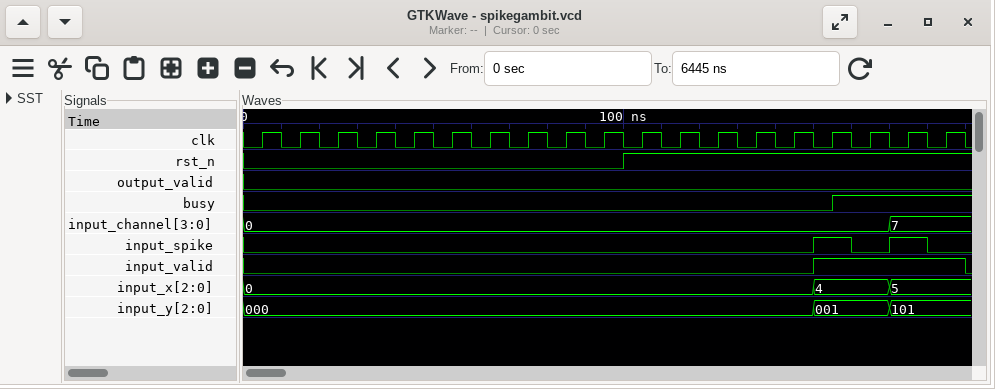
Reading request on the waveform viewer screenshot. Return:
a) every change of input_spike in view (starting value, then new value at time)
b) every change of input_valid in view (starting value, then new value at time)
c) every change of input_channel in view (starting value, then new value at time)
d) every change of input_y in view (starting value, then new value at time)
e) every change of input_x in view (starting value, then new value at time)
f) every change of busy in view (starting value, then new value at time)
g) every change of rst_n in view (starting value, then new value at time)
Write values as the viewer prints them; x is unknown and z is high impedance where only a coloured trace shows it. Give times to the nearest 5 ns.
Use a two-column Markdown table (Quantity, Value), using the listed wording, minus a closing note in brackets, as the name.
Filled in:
| Quantity | Value |
|---|---|
| every change of input_spike in view | 0, 1 at 150 ns, 0 at 160 ns, 1 at 170 ns, 0 at 180 ns |
| every change of input_valid in view | 0, 1 at 150 ns, 0 at 190 ns |
| every change of input_channel in view | 0, 7 at 170 ns |
| every change of input_y in view | 000, 001 at 150 ns, 101 at 170 ns |
| every change of input_x in view | 0, 4 at 150 ns, 5 at 170 ns |
| every change of busy in view | 0, 1 at 155 ns |
| every change of rst_n in view | 0, 1 at 100 ns |
